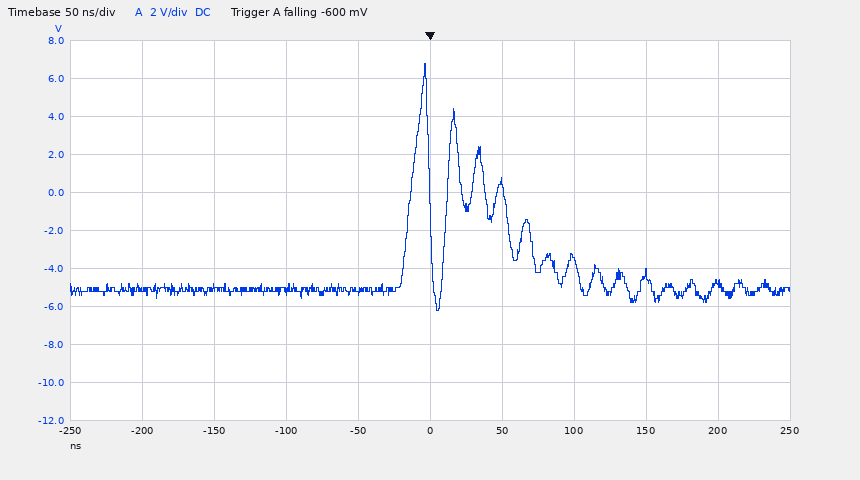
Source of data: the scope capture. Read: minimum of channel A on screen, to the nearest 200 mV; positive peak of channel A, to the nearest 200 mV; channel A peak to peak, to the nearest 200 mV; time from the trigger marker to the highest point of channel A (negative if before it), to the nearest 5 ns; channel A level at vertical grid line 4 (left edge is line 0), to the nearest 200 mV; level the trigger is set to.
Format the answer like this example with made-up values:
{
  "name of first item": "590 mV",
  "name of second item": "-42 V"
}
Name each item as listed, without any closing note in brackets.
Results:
{
  "minimum of channel A on screen, to the nearest 200 mV": "-6.2 V",
  "positive peak of channel A, to the nearest 200 mV": "6.8 V",
  "channel A peak to peak, to the nearest 200 mV": "13.0 V",
  "time from the trigger marker to the highest point of channel A (negative if before it), to the nearest 5 ns": "-5 ns",
  "channel A level at vertical grid line 4 (left edge is line 0), to the nearest 200 mV": "-5.2 V",
  "level the trigger is set to": "-600 mV"
}
